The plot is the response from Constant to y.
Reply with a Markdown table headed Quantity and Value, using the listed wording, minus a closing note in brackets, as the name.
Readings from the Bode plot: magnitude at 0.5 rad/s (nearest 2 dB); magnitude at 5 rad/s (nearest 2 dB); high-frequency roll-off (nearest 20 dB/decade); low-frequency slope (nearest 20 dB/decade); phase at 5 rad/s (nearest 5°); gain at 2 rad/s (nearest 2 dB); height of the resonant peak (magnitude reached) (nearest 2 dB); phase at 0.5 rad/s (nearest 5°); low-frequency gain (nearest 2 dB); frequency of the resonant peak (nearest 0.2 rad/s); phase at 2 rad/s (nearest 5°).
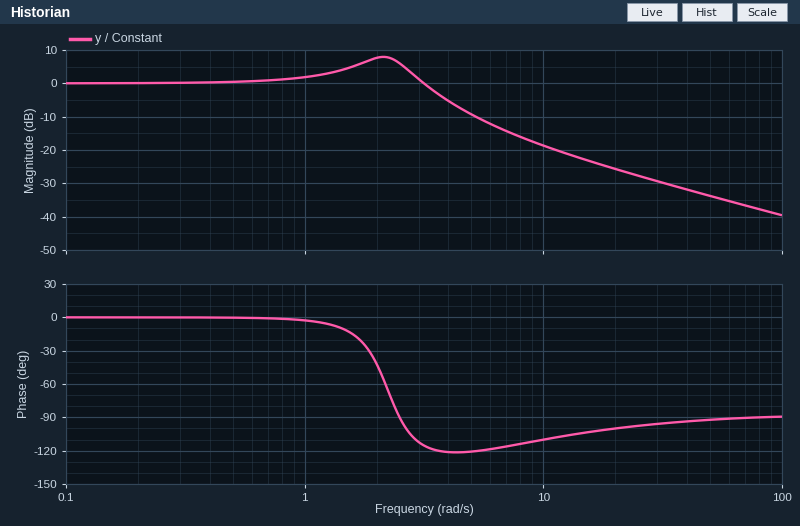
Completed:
| Quantity | Value |
|---|---|
| magnitude at 0.5 rad/s | 0 dB |
| magnitude at 5 rad/s | -10 dB |
| high-frequency roll-off | -20 dB/decade |
| low-frequency slope | 0 dB/decade |
| phase at 5 rad/s | -120° |
| gain at 2 rad/s | 8 dB |
| height of the resonant peak (magnitude reached) | 8 dB |
| phase at 0.5 rad/s | 0° |
| low-frequency gain | 0 dB |
| frequency of the resonant peak | 2.2 rad/s |
| phase at 2 rad/s | -40° |
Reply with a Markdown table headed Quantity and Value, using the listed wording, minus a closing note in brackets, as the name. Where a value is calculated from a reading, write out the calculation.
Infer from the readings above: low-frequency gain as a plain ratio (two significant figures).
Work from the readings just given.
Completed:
| Quantity | Value |
|---|---|
| low-frequency gain as a plain ratio | 10^(0 / 20) = 1.0 |
